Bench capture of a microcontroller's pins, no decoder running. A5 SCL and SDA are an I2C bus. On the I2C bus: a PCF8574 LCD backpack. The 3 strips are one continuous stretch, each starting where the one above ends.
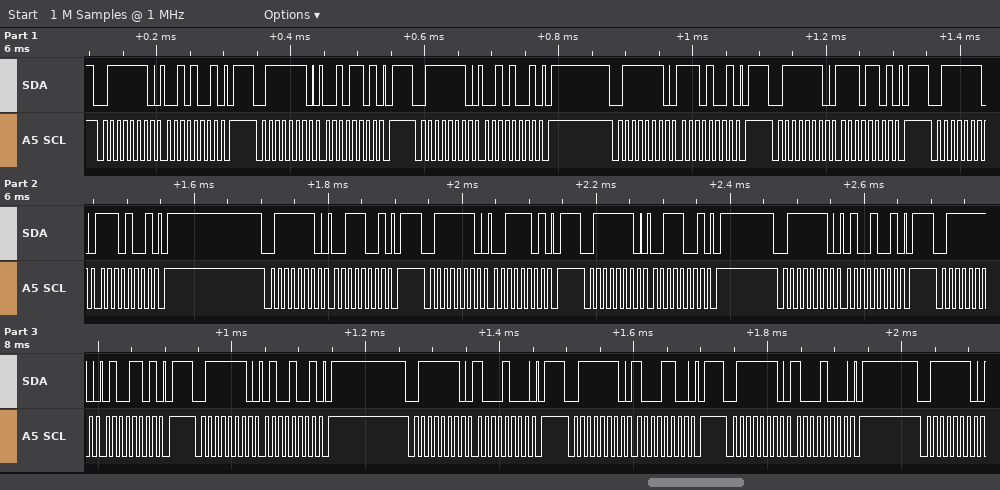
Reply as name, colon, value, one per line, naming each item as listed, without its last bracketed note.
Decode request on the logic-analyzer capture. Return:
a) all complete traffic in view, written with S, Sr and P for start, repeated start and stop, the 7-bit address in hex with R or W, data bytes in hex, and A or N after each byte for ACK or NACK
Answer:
all complete traffic in view, written with S, Sr and P for start, repeated start and stop, the 7-bit address in hex with R or W, data bytes in hex, and A or N after each byte for ACK or NACK: S 3FW A 29 A P S 3FW A 2D A P S 3FW A 29 A P S 3FW A E9 A P S 3FW A ED A P S 3FW A E9 A P S 3FW A 39 A P S 3FW A 3D A P S 3FW A 39 A P S 3FW A 49 A P S 3FW A 4D A P S 3FW A 49 A P S 3FW A 88 A P S 3FW A 8C A P S 3FW A 88 A P S 3FW A
